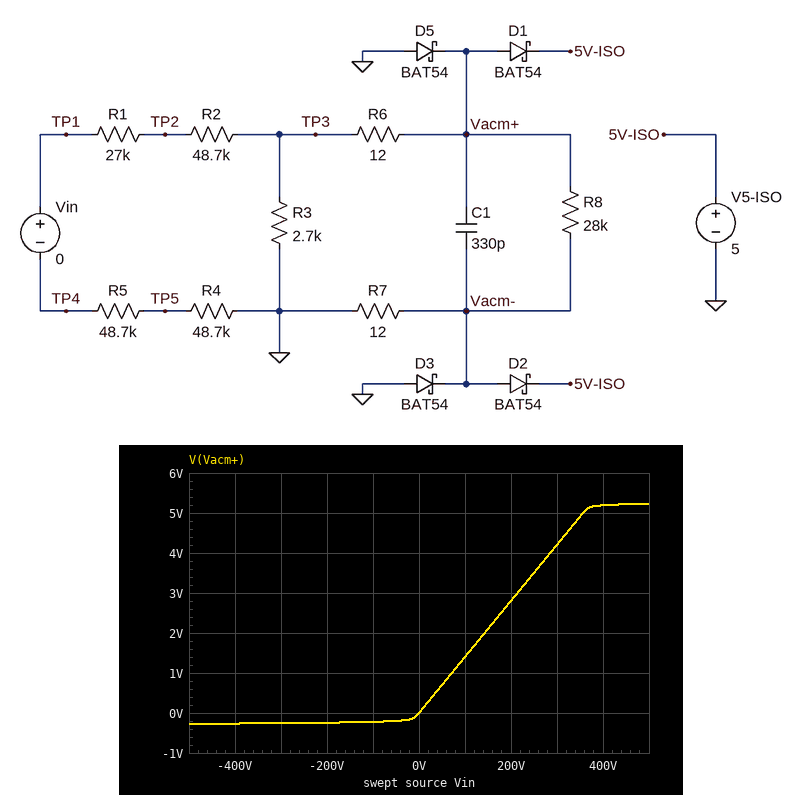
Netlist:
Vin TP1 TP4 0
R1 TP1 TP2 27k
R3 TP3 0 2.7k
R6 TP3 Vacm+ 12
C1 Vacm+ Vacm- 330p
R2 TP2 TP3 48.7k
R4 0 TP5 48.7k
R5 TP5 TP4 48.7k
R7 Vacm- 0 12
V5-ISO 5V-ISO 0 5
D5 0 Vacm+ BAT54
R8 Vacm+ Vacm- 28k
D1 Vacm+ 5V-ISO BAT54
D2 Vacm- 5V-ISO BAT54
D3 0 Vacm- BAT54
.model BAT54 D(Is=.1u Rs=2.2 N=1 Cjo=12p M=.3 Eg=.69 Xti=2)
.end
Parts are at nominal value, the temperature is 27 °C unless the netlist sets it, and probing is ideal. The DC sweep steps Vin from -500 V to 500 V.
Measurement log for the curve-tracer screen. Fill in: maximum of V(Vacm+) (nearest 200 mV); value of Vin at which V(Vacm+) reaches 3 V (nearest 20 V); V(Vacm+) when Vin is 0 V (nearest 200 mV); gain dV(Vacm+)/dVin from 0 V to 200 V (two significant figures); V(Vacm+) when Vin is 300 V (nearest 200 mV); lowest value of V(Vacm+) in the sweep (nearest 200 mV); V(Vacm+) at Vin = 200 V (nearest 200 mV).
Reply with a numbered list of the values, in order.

1. 5.2 V
2. 220 V
3. 0 V
4. 0.014 V/V
5. 4.2 V
6. -200 mV
7. 2.8 V
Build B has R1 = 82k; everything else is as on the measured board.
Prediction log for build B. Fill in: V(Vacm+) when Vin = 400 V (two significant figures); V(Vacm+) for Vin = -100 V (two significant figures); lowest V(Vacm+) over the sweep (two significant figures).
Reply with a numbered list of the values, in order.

1. 4.3 V
2. -210 mV
3. -260 mV
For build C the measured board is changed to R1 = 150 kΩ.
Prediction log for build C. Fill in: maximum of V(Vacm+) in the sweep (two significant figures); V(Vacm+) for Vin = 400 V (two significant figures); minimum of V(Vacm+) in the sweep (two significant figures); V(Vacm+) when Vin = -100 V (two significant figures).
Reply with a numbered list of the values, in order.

1. 4.1 V
2. 3.3 V
3. -250 mV
4. -200 mV
